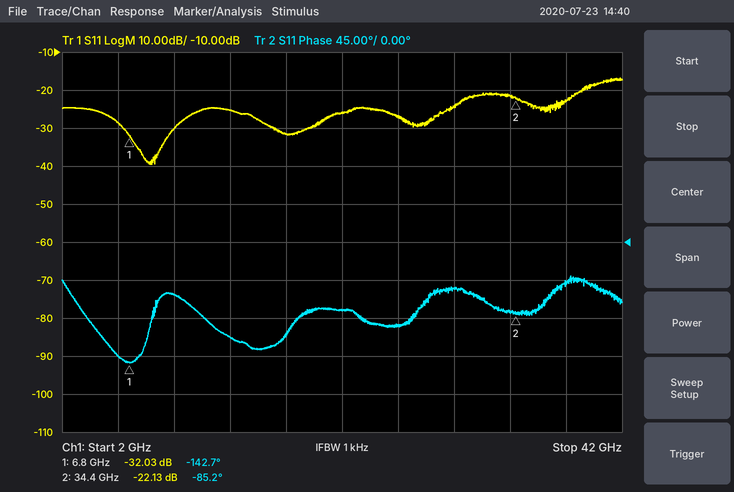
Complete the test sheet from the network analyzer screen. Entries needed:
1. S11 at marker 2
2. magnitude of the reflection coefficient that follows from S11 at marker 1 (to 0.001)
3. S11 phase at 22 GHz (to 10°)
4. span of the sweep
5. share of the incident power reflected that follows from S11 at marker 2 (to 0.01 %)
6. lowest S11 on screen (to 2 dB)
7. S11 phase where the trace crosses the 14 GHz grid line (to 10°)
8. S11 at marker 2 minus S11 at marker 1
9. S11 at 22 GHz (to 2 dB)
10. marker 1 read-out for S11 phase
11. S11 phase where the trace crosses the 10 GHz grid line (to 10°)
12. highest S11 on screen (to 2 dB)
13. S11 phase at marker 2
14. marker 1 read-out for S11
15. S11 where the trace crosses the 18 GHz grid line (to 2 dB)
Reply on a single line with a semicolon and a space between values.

-22.13 dB; 0.025; -80°; 40 GHz; 0.61 %; -40 dB; -110°; 9.90 dB; -26 dB; -142.7°; -60°; -16 dB; -85.2°; -32.03 dB; -32 dB
